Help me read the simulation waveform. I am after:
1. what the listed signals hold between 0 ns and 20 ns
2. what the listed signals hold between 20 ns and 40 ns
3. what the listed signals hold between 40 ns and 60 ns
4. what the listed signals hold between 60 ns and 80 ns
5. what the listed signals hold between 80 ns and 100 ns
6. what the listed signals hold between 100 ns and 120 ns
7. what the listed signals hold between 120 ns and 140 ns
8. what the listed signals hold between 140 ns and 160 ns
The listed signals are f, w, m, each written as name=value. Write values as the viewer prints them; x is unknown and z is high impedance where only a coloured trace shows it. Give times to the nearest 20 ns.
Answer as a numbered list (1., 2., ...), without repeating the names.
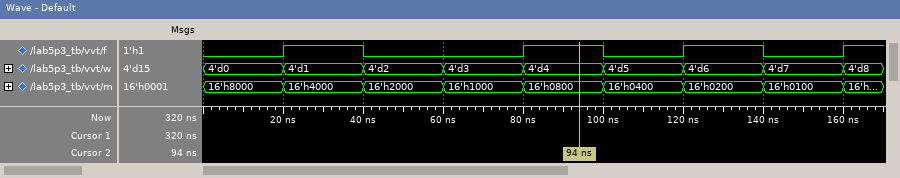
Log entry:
1. f=0, w=4'd0, m=16'h8000
2. f=1, w=4'd1, m=16'h4000
3. f=0, w=4'd2, m=16'h2000
4. f=0, w=4'd3, m=16'h1000
5. f=1, w=4'd4, m=16'h0800
6. f=0, w=4'd5, m=16'h0400
7. f=1, w=4'd6, m=16'h0200
8. f=0, w=4'd7, m=16'h0100
